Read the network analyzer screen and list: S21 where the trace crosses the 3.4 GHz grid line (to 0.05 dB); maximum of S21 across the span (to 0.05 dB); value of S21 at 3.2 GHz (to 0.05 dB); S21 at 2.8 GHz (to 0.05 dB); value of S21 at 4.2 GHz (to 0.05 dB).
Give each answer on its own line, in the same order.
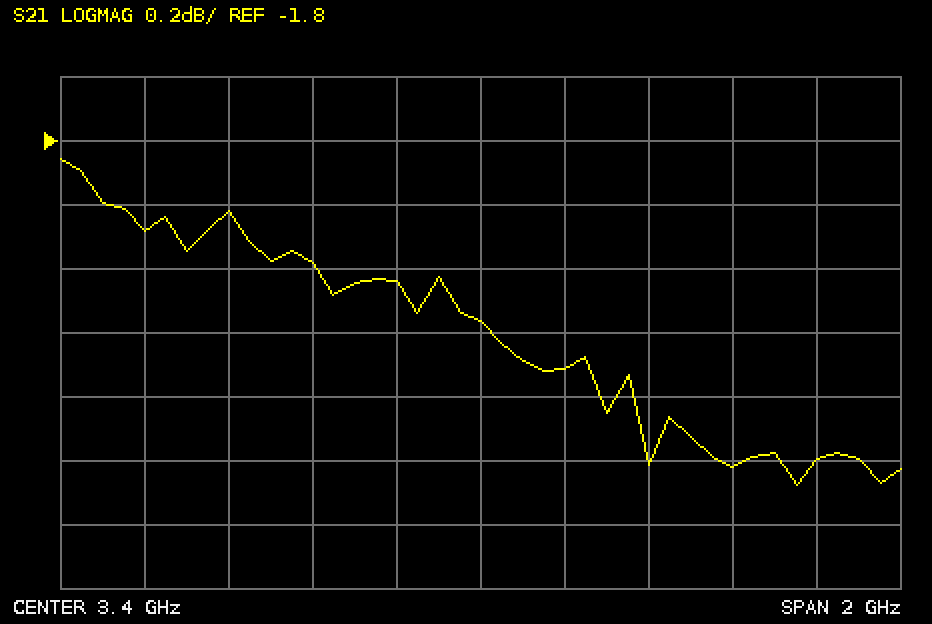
-2.35 dB
-1.85 dB
-2.25 dB
-2.00 dB
-2.80 dB
